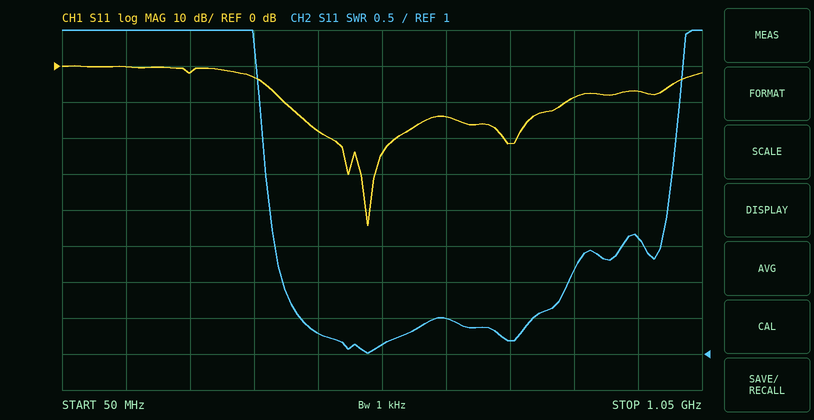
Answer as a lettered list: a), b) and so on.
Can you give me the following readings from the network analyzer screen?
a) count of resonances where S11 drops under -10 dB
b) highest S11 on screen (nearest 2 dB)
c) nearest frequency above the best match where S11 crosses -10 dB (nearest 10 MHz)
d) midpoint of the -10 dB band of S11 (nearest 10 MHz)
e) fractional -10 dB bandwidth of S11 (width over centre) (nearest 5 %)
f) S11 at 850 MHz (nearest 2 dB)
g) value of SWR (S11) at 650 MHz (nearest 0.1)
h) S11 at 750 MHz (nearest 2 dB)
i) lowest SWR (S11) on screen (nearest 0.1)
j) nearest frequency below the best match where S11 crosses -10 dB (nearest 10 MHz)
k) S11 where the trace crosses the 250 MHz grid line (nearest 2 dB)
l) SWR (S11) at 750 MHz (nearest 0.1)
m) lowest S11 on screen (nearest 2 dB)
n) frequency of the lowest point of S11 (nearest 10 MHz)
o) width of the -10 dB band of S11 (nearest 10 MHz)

a) 3
b) 0 dB
c) 840 MHz
d) 620 MHz
e) 70 %
f) -8 dB
g) 1.5
h) -22 dB
i) 1.0
j) 400 MHz
k) -2 dB
l) 1.2
m) -44 dB
n) 530 MHz
o) 440 MHz
